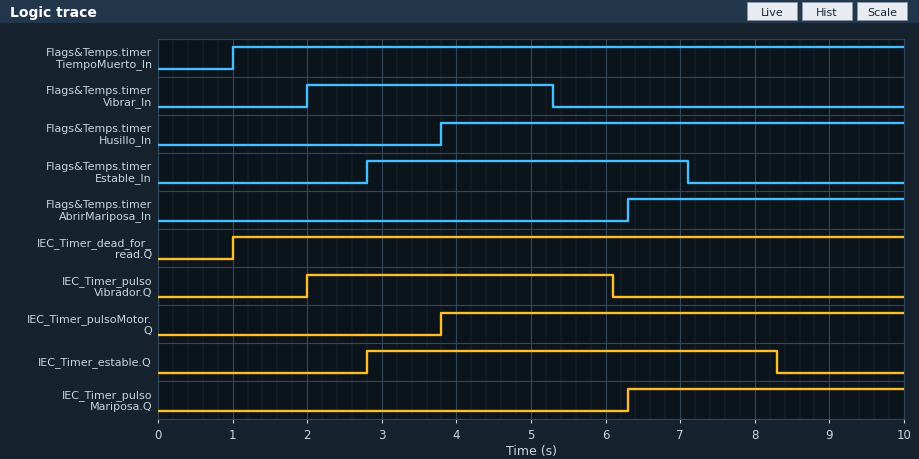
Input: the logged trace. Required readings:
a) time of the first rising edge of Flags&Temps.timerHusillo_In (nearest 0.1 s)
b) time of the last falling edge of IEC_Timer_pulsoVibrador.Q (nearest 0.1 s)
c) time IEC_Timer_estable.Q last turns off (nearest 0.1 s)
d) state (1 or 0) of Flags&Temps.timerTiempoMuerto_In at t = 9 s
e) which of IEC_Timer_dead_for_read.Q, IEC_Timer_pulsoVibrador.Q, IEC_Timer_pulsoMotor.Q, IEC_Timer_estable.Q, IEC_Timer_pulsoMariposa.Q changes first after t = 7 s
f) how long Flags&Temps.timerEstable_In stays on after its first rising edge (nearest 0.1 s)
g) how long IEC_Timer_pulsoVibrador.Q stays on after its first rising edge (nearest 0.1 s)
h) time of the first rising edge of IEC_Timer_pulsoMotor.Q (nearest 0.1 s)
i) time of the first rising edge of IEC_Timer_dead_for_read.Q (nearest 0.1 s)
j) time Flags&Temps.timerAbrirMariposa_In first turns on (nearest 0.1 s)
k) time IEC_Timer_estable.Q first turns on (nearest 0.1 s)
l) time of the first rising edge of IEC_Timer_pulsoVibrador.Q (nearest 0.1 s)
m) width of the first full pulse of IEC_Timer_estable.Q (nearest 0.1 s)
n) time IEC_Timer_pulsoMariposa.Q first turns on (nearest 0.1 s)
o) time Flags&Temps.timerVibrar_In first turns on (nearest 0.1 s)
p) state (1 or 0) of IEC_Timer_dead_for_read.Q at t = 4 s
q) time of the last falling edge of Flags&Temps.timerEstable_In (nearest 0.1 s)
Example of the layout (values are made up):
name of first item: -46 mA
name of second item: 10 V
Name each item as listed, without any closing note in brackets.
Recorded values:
time of the first rising edge of Flags&Temps.timerHusillo_In: 3.8 s
time of the last falling edge of IEC_Timer_pulsoVibrador.Q: 6.1 s
time IEC_Timer_estable.Q last turns off: 8.3 s
state (1 or 0) of Flags&Temps.timerTiempoMuerto_In at t = 9 s: 1
which of IEC_Timer_dead_for_read.Q, IEC_Timer_pulsoVibrador.Q, IEC_Timer_pulsoMotor.Q, IEC_Timer_estable.Q, IEC_Timer_pulsoMariposa.Q changes first after t = 7 s: IEC_Timer_estable.Q
how long Flags&Temps.timerEstable_In stays on after its first rising edge: 4.3 s
how long IEC_Timer_pulsoVibrador.Q stays on after its first rising edge: 4.1 s
time of the first rising edge of IEC_Timer_pulsoMotor.Q: 3.8 s
time of the first rising edge of IEC_Timer_dead_for_read.Q: 1.0 s
time Flags&Temps.timerAbrirMariposa_In first turns on: 6.3 s
time IEC_Timer_estable.Q first turns on: 2.8 s
time of the first rising edge of IEC_Timer_pulsoVibrador.Q: 2.0 s
width of the first full pulse of IEC_Timer_estable.Q: 5.5 s
time IEC_Timer_pulsoMariposa.Q first turns on: 6.3 s
time Flags&Temps.timerVibrar_In first turns on: 2.0 s
state (1 or 0) of IEC_Timer_dead_for_read.Q at t = 4 s: 1
time of the last falling edge of Flags&Temps.timerEstable_In: 7.1 s
